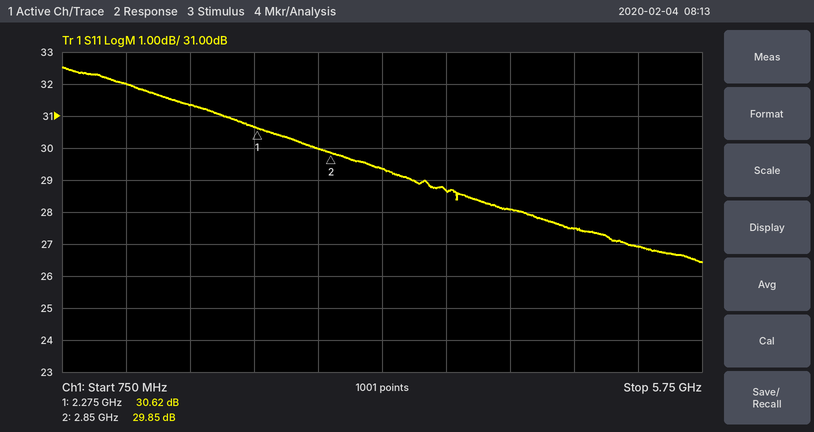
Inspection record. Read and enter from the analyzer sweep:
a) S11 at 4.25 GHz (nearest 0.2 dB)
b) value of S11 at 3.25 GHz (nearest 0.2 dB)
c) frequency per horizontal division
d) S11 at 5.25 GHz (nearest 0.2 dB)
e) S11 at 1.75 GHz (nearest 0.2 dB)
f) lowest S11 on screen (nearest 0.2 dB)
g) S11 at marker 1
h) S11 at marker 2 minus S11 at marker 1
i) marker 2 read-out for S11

28.0 dB
29.4 dB
500 MHz
27.0 dB
31.4 dB
26.4 dB
30.62 dB
-0.77 dB
29.85 dB
